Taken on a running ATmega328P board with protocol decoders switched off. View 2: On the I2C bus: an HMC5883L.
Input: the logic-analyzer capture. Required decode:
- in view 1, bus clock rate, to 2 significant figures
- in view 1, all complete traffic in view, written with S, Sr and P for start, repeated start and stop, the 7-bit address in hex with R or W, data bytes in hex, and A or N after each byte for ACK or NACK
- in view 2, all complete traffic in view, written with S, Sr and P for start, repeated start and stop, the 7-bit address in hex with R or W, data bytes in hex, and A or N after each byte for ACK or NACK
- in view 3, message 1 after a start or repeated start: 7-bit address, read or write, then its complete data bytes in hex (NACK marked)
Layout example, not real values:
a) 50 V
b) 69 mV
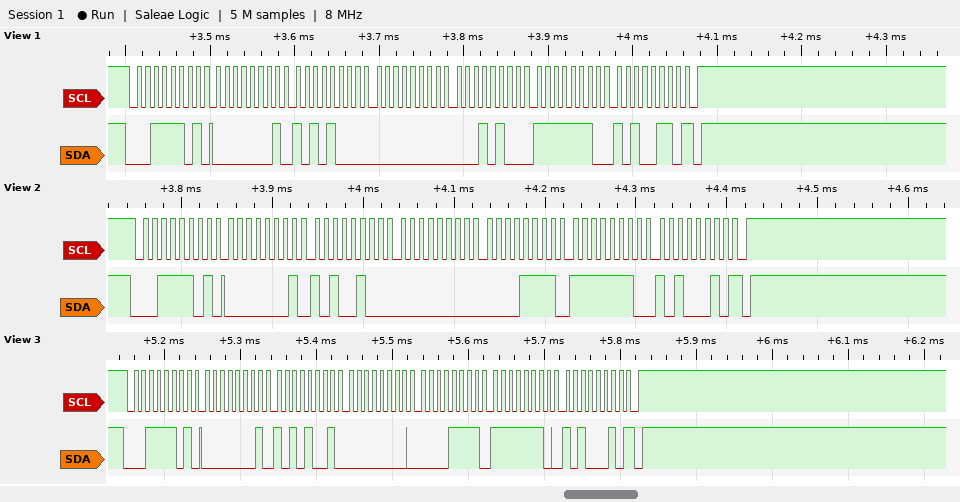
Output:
a) 100 kHz
b) S 1ER A 01 A A8 A 00 A 14 A FE A A6 N P
c) S 1ER A 01 A A4 A 00 A 0F A FE A A2 N P
d) 0x1E read: 01 A9 00 0F FE A2 NACK
